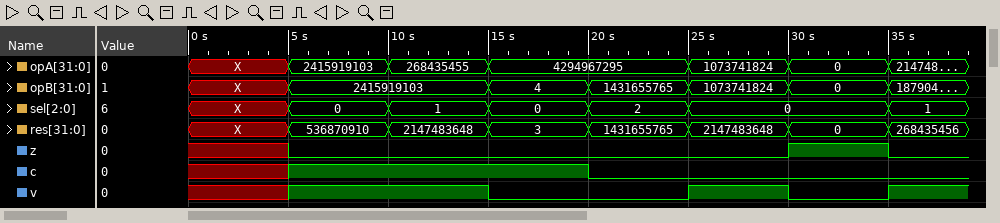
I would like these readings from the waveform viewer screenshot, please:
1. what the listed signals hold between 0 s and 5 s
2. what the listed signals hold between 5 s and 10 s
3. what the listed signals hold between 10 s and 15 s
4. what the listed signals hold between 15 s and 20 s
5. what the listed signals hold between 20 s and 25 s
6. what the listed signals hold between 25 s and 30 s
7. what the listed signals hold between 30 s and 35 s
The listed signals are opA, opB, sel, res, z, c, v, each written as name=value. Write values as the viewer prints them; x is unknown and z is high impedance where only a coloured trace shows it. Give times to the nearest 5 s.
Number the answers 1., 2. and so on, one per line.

1. opA=X, opB=X, sel=X, res=X, z=x, c=x, v=x
2. opA=2415919103, opB=2415919103, sel=0, res=536870910, z=0, c=1, v=1
3. opA=268435455, opB=2415919103, sel=1, res=2147483648, z=0, c=1, v=1
4. opA=4294967295, opB=4, sel=0, res=3, z=0, c=1, v=0
5. opA=4294967295, opB=1431655765, sel=2, res=1431655765, z=0, c=0, v=0
6. opA=1073741824, opB=1073741824, sel=0, res=2147483648, z=0, c=0, v=1
7. opA=0, opB=0, sel=0, res=0, z=1, c=0, v=0
